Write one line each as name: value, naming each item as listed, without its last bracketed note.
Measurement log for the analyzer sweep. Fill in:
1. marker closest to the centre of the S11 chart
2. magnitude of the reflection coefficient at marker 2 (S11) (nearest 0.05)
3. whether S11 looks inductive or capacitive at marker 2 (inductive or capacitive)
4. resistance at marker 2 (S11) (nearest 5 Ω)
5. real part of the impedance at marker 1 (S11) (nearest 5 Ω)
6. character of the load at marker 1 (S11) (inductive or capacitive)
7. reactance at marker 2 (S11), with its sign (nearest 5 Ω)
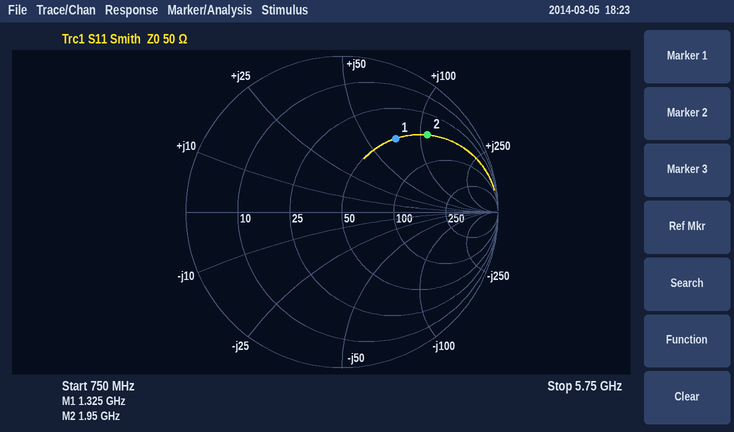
marker closest to the centre of the S11 chart: marker 1
magnitude of the reflection coefficient at marker 2 (S11): 0.75
whether S11 looks inductive or capacitive at marker 2: inductive
resistance at marker 2 (S11): 50 Ω
real part of the impedance at marker 1 (S11): 50 Ω
character of the load at marker 1 (S11): inductive
reactance at marker 2 (S11), with its sign: +110 Ω
